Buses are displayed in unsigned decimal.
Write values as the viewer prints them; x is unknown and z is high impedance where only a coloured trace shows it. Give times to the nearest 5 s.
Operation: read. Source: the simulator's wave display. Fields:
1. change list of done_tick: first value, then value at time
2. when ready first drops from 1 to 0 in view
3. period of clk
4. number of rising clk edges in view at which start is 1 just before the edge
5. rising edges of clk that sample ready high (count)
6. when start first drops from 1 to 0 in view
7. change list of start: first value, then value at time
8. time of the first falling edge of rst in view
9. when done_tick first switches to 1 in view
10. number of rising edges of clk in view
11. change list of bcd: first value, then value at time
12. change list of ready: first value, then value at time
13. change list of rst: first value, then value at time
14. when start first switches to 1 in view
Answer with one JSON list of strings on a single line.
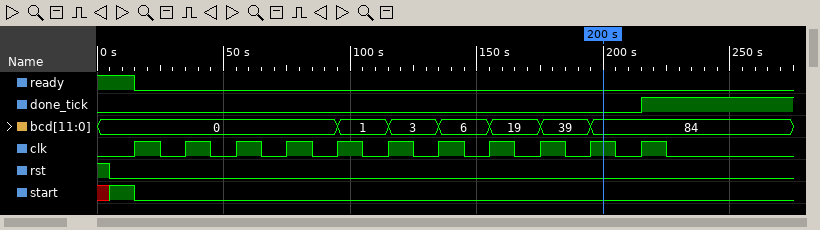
["0, 1 at 215 s", "15 s", "20 s", "1", "1", "15 s", "x, 1 at 5 s, 0 at 15 s", "5 s", "215 s", "11", "0, 1 at 95 s, 3 at 115 s, 6 at 135 s, 19 at 155 s, 39 at 175 s, 84 at 195 s", "1, 0 at 15 s", "1, 0 at 5 s", "5 s"]
